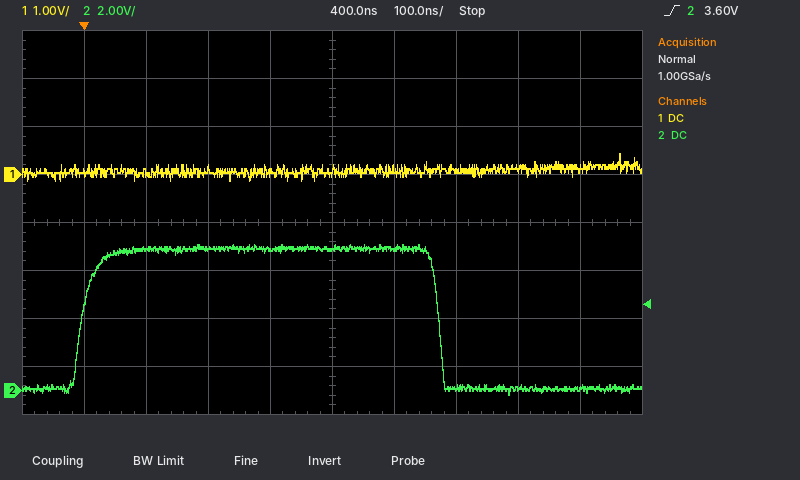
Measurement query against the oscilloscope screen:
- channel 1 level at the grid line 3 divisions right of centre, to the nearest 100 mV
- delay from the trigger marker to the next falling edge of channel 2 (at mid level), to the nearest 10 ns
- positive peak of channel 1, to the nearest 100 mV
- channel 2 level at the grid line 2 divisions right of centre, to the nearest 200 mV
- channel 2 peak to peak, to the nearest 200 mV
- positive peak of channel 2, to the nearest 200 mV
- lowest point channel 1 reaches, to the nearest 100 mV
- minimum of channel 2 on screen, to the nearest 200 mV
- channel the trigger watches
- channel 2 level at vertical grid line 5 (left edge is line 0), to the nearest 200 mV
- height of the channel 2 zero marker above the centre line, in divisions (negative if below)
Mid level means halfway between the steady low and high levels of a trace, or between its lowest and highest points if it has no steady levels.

100 mV
570 ns
400 mV
200 mV
6.2 V
6.0 V
-100 mV
-200 mV
channel 2
6.0 V
-3.5 div
